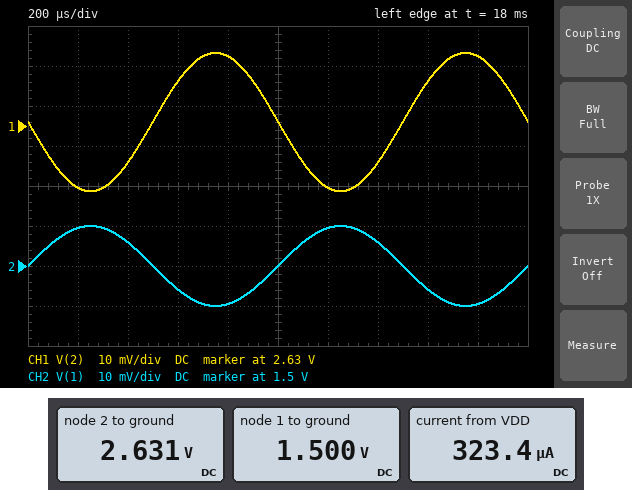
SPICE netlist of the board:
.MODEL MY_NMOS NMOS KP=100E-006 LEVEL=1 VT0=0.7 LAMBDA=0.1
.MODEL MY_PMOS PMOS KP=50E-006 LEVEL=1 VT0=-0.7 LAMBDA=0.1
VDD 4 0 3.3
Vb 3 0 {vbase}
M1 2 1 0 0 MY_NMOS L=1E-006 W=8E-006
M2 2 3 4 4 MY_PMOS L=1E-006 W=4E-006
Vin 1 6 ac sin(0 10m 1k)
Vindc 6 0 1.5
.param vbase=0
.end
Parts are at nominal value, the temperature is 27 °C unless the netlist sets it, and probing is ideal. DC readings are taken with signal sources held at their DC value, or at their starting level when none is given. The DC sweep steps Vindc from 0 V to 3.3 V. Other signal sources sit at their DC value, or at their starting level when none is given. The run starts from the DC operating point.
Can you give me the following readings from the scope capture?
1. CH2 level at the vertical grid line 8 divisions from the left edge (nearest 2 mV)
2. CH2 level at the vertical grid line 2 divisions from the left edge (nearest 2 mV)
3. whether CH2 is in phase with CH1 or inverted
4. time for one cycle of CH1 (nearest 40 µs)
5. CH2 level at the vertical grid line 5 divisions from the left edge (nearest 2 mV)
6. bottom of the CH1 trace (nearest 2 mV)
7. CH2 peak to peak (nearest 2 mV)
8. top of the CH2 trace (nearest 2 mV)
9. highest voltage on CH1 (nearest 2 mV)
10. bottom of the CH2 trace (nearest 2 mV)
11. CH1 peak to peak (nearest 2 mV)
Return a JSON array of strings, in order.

["1.494 V", "1.506 V", "inverted", "1.00 ms", "1.500 V", "2.614 V", "20 mV", "1.510 V", "2.648 V", "1.490 V", "34 mV"]
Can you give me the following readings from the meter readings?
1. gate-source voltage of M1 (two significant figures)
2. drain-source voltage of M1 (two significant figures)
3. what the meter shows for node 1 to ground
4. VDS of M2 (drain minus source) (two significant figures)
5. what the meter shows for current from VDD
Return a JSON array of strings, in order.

["1.5 V", "2.6 V", "1.500 V", "-670 mV", "323.4 µA"]
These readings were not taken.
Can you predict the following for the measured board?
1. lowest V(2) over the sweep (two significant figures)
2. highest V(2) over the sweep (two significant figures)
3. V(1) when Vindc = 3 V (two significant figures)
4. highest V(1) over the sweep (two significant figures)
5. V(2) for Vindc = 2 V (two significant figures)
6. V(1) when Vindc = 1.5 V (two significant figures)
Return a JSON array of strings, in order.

["440 mV", "3.3 V", "3.0 V", "3.3 V", "1.3 V", "1.5 V"]
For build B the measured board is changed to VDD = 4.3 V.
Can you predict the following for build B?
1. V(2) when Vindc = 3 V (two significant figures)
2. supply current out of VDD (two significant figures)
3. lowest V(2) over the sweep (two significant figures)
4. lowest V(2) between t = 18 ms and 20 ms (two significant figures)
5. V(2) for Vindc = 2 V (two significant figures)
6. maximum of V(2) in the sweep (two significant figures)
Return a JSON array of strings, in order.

["1.1 V", "350 µA", "920 mV", "3.8 V", "3.0 V", "4.3 V"]
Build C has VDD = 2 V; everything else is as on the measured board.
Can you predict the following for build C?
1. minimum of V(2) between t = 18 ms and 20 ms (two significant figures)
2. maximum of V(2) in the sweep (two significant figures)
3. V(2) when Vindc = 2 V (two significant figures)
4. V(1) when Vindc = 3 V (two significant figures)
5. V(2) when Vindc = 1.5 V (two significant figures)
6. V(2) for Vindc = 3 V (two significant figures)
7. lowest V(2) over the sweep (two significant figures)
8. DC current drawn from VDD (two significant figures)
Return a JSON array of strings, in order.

["380 mV", "2.0 V", "200 mV", "3.0 V", "390 mV", "110 mV", "98 mV", "200 µA"]
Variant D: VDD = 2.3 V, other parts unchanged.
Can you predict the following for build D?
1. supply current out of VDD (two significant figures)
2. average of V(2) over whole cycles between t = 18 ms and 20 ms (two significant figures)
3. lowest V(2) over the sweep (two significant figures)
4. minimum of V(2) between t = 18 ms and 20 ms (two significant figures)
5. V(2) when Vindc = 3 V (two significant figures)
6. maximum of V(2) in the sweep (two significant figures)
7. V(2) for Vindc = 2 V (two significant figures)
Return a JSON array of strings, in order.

["280 µA", "980 mV", "150 mV", "910 mV", "170 mV", "2.3 V", "330 mV"]
